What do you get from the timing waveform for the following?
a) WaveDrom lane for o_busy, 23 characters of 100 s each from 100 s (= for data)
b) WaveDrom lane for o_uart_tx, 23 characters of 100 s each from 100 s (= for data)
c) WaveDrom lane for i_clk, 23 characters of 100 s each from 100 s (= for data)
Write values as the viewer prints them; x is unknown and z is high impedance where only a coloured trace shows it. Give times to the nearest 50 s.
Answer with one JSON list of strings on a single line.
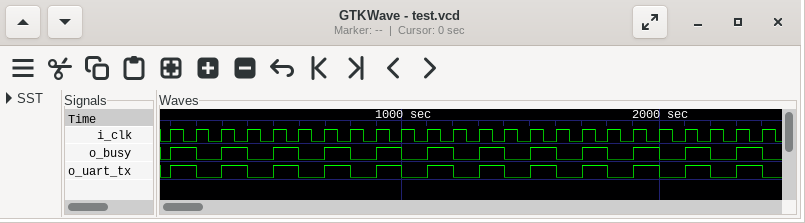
["{name: 'o_busy', wave: '10101010101010101010101'}", "{name: 'o_uart_tx', wave: '10101010101010101010101'}", "{name: 'i_clk', wave: 'p......................'}"]
